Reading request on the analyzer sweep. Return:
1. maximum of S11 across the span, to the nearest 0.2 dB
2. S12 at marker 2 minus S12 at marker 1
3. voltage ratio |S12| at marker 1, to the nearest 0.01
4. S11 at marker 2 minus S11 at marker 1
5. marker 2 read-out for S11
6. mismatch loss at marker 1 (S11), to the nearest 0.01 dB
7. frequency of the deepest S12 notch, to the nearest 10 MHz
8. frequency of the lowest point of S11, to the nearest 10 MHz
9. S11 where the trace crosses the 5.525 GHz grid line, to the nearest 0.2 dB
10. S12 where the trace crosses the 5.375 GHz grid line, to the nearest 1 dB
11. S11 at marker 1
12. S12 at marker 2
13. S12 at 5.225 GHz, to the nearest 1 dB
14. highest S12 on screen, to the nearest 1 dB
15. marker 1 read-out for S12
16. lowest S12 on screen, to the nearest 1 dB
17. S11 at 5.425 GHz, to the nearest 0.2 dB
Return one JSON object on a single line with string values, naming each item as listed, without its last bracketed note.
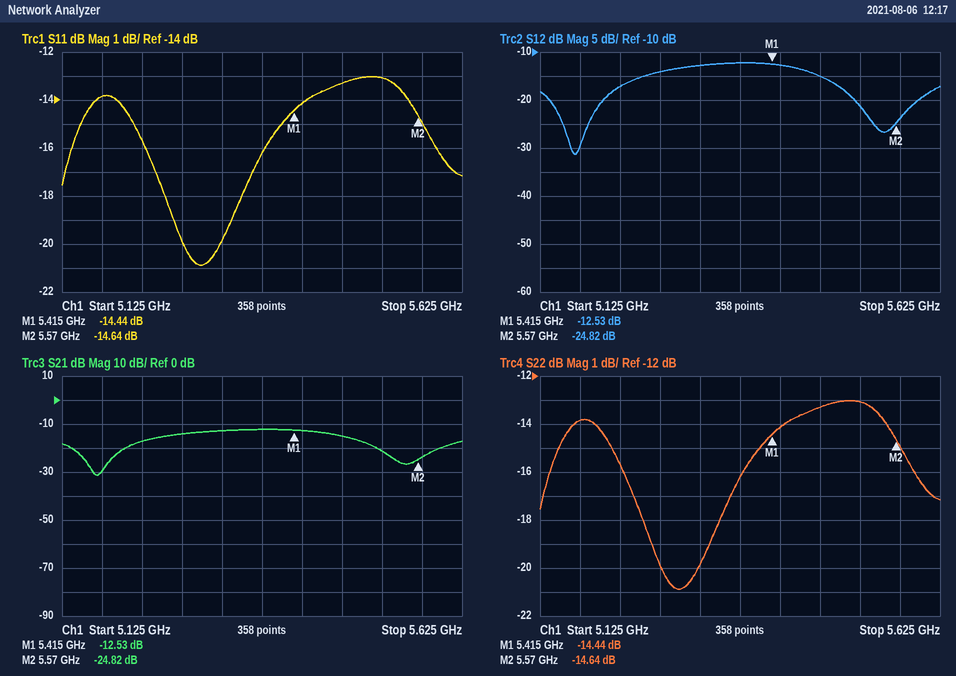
{"maximum of S11 across the span, to the nearest 0.2 dB": "-13.0 dB", "S12 at marker 2 minus S12 at marker 1": "-12.29 dB", "voltage ratio |S12| at marker 1, to the nearest 0.01": "0.24", "S11 at marker 2 minus S11 at marker 1": "-0.20 dB", "marker 2 read-out for S11": "-14.64 dB", "mismatch loss at marker 1 (S11), to the nearest 0.01 dB": "0.16 dB", "frequency of the deepest S12 notch, to the nearest 10 MHz": "5.17 GHz", "frequency of the lowest point of S11, to the nearest 10 MHz": "5.30 GHz", "S11 where the trace crosses the 5.525 GHz grid line, to the nearest 0.2 dB": "-13.0 dB", "S12 where the trace crosses the 5.375 GHz grid line, to the nearest 1 dB": "-12 dB", "S11 at marker 1": "-14.44 dB", "S12 at marker 2": "-24.82 dB", "S12 at 5.225 GHz, to the nearest 1 dB": "-17 dB", "highest S12 on screen, to the nearest 1 dB": "-12 dB", "marker 1 read-out for S12": "-12.53 dB", "lowest S12 on screen, to the nearest 1 dB": "-31 dB", "S11 at 5.425 GHz, to the nearest 0.2 dB": "-14.2 dB"}
